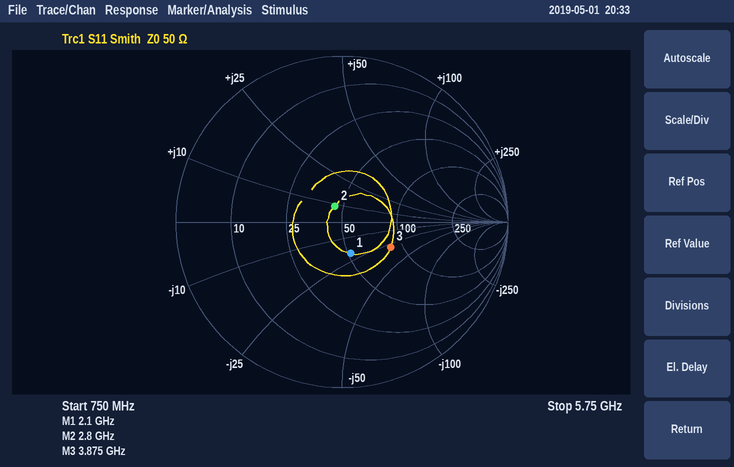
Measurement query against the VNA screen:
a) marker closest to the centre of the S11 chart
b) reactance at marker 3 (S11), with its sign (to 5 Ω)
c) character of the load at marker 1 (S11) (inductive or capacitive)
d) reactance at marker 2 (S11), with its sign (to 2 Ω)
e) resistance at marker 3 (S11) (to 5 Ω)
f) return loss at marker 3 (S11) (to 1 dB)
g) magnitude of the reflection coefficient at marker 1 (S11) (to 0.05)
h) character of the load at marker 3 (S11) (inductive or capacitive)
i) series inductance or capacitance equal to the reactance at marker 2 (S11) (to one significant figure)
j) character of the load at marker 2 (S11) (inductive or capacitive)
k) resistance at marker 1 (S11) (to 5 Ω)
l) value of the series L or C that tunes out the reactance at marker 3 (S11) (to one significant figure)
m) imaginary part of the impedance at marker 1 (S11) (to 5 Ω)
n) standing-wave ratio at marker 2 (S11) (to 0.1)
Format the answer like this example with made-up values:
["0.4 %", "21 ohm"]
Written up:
["marker 2", "-30 Ω", "capacitive", "+8 Ω", "85 Ω", "10 dB", "0.20", "capacitive", "500 pH", "inductive", "50 Ω", "1 nH", "-20 Ω", "1.2"]
